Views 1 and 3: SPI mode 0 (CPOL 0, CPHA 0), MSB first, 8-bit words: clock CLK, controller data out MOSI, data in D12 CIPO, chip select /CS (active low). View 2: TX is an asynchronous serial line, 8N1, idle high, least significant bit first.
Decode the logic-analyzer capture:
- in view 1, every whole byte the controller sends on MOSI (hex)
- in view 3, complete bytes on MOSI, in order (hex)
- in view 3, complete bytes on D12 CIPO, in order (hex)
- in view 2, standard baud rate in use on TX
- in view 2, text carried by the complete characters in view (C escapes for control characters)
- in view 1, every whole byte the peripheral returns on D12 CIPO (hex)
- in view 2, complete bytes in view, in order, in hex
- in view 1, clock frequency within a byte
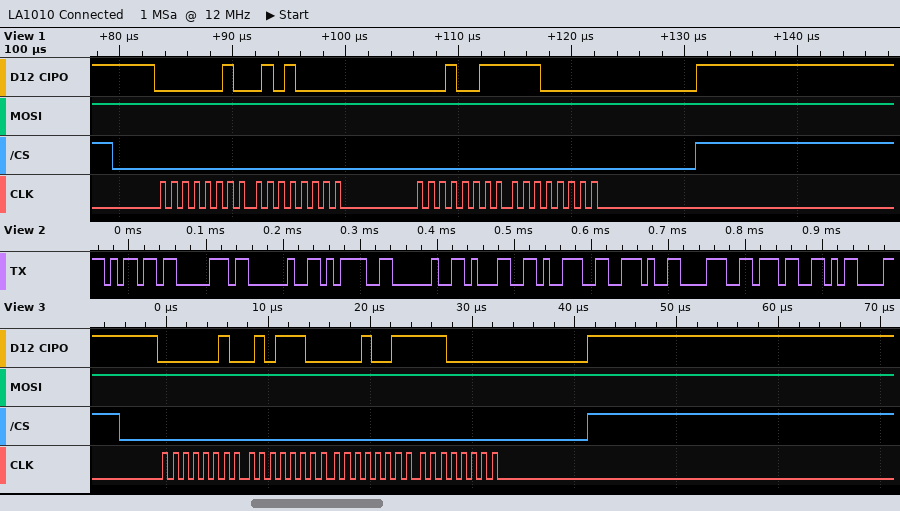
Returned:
FF FF FF FF
FF FF FF FF
02 5C 13 E0
115200 baud
"mp = 19.87\r"
02 50 13 E0
6D 70 20 3D 20 31 39 2E 38 37 0D
1 MHz
